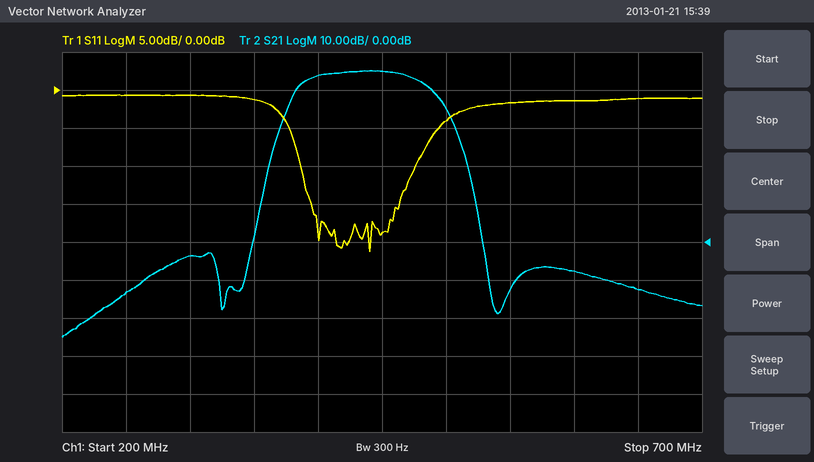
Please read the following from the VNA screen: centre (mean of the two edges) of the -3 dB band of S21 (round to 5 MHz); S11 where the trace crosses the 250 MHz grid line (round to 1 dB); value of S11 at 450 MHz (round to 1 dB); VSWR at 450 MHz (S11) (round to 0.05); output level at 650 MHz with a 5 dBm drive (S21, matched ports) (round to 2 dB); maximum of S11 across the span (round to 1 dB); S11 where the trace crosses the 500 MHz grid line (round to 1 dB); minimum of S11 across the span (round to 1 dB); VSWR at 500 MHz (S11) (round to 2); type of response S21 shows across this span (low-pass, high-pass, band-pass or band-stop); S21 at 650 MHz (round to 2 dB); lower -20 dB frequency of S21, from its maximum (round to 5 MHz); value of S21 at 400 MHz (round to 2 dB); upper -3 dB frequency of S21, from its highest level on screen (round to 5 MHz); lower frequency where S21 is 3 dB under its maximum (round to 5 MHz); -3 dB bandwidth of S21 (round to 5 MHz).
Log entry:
435 MHz
-1 dB
-19 dB
1.25
-8 dBm
-1 dB
-4 dB
-21 dB
4
band-pass
-12 dB
365 MHz
44 dB
480 MHz
390 MHz
90 MHz
